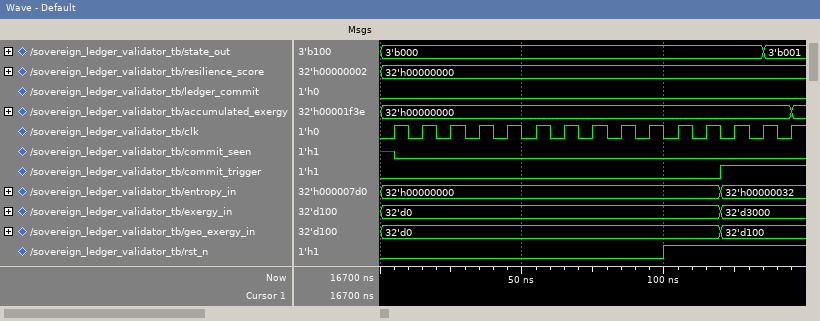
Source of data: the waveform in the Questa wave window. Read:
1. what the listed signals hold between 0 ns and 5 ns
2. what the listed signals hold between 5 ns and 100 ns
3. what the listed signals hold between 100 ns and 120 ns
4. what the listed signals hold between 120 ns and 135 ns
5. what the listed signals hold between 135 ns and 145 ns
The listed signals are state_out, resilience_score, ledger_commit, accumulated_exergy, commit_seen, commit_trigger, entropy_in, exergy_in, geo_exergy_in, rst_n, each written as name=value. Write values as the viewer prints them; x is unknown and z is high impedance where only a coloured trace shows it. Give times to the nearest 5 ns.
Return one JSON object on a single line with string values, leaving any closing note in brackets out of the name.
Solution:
{"what the listed signals hold between 0 ns and 5 ns": "state_out=3'b000, resilience_score=32'h00000000, ledger_commit=0, accumulated_exergy=32'h00000000, commit_seen=x, commit_trigger=0, entropy_in=32'h00000000, exergy_in=32'd0, geo_exergy_in=32'd0, rst_n=0", "what the listed signals hold between 5 ns and 100 ns": "state_out=3'b000, resilience_score=32'h00000000, ledger_commit=0, accumulated_exergy=32'h00000000, commit_seen=0, commit_trigger=0, entropy_in=32'h00000000, exergy_in=32'd0, geo_exergy_in=32'd0, rst_n=0", "what the listed signals hold between 100 ns and 120 ns": "state_out=3'b000, resilience_score=32'h00000000, ledger_commit=0, accumulated_exergy=32'h00000000, commit_seen=0, commit_trigger=0, entropy_in=32'h00000000, exergy_in=32'd0, geo_exergy_in=32'd0, rst_n=1", "what the listed signals hold between 120 ns and 135 ns": "state_out=3'b000, resilience_score=32'h00000000, ledger_commit=0, accumulated_exergy=32'h00000000, commit_seen=0, commit_trigger=1, entropy_in=32'h00000032, exergy_in=32'd3000, geo_exergy_in=32'd100, rst_n=1", "what the listed signals hold between 135 ns and 145 ns": "state_out=3'b001, resilience_score=32'h00000000, ledger_commit=0, accumulated_exergy=32'h00000000, commit_seen=0, commit_trigger=1, entropy_in=32'h00000032, exergy_in=32'd3000, geo_exergy_in=32'd100, rst_n=1"}
